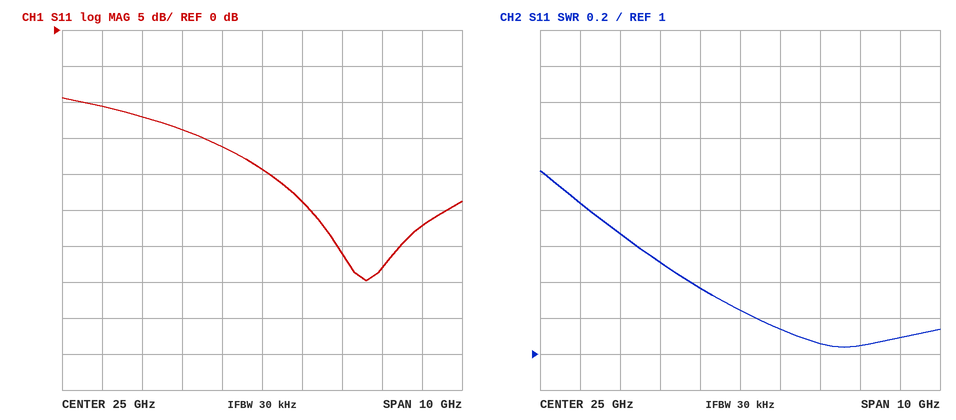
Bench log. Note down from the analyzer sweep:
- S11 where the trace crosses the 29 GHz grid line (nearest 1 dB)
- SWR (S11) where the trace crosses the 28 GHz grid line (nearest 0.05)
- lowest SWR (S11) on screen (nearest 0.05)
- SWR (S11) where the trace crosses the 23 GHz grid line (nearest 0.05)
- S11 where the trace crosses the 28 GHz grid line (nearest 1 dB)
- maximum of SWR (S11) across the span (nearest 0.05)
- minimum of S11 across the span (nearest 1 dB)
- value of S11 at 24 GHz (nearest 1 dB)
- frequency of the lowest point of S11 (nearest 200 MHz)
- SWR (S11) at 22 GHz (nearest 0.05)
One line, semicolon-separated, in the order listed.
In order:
-27 dB; 1.05; 1.05; 1.50; -33 dB; 2.00; -35 dB; -16 dB; 27.6 GHz; 1.65
